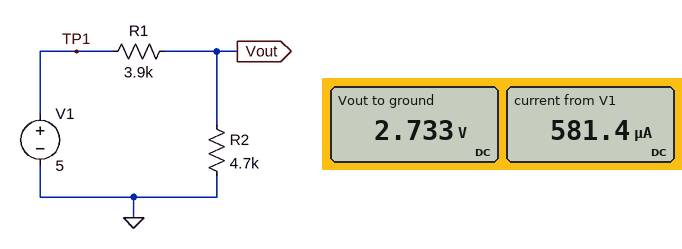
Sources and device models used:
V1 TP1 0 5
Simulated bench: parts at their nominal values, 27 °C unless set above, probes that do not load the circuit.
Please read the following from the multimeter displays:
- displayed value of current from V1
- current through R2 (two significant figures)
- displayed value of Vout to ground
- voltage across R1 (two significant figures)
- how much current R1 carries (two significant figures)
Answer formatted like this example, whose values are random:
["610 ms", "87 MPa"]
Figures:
["581.4 µA", "580 µA", "2.733 V", "2.3 V", "580 µA"]
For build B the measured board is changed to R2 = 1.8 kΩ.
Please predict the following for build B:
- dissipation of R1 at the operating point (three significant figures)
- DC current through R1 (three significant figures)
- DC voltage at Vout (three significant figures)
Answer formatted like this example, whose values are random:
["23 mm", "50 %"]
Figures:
["3.00 mW", "877 µA", "1.58 V"]
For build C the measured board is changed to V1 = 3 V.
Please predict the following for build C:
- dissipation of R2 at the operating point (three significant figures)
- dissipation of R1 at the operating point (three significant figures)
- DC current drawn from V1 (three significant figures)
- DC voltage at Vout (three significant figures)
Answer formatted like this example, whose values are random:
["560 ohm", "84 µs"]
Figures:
["572 µW", "475 µW", "349 µA", "1.64 V"]
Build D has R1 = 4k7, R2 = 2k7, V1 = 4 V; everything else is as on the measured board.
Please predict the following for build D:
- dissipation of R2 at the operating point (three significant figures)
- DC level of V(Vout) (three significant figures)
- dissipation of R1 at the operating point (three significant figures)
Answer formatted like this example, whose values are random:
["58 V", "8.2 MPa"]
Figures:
["789 µW", "1.46 V", "1.37 mW"]
